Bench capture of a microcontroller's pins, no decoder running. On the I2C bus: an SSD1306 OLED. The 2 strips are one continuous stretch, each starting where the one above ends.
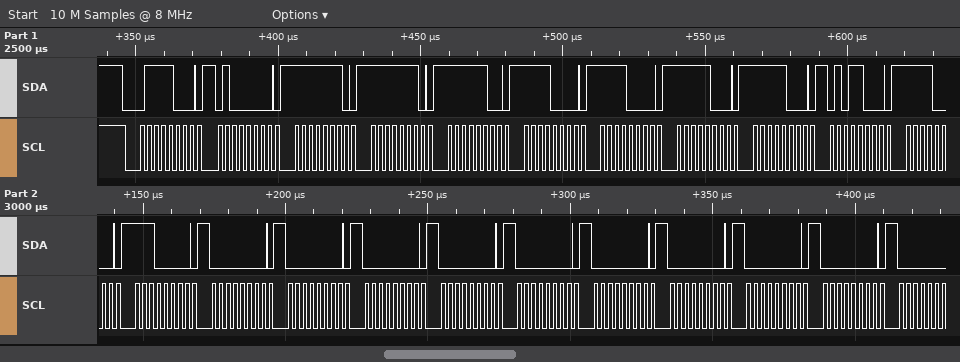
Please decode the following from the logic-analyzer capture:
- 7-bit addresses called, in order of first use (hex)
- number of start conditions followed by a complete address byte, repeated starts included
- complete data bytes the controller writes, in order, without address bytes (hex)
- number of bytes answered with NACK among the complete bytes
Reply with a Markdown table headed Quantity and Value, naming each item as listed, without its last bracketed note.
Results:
| Quantity | Value |
|---|---|
| 7-bit addresses called, in order of first use | 0x3C |
| number of start conditions followed by a complete address byte, repeated starts included | 1 |
| complete data bytes the controller writes, in order, without address bytes | 40 FE FE FC F0 F0 F8 F8 58 F0 E0 00 00 00 00 00 00 00 00 00 |
| number of bytes answered with NACK among the complete bytes | 0 |
